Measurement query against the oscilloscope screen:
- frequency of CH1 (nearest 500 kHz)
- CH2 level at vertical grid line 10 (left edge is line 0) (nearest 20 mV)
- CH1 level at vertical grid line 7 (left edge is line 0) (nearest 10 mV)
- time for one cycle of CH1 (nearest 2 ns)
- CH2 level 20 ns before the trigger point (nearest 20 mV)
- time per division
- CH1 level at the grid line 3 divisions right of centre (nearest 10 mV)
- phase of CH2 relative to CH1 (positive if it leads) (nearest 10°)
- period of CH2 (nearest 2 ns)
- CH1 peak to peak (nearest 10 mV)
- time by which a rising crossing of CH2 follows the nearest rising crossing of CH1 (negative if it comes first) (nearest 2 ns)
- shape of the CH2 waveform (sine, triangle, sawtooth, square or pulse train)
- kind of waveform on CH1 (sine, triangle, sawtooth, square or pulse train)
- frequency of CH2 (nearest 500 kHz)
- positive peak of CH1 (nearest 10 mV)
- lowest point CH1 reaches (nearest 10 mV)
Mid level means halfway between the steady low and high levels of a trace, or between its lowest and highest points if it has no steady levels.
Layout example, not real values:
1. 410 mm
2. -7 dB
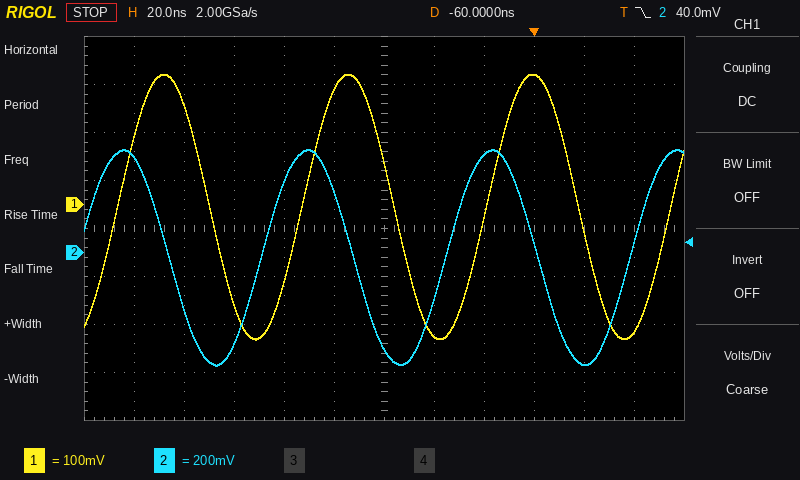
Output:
1. 13.5 MHz
2. -460 mV
3. -270 mV
4. 74 ns
5. 400 mV
6. 20 ns
7. 270 mV
8. +80°
9. 74 ns
10. 550 mV
11. -16 ns
12. sine
13. sine
14. 13.5 MHz
15. 270 mV
16. -280 mV
